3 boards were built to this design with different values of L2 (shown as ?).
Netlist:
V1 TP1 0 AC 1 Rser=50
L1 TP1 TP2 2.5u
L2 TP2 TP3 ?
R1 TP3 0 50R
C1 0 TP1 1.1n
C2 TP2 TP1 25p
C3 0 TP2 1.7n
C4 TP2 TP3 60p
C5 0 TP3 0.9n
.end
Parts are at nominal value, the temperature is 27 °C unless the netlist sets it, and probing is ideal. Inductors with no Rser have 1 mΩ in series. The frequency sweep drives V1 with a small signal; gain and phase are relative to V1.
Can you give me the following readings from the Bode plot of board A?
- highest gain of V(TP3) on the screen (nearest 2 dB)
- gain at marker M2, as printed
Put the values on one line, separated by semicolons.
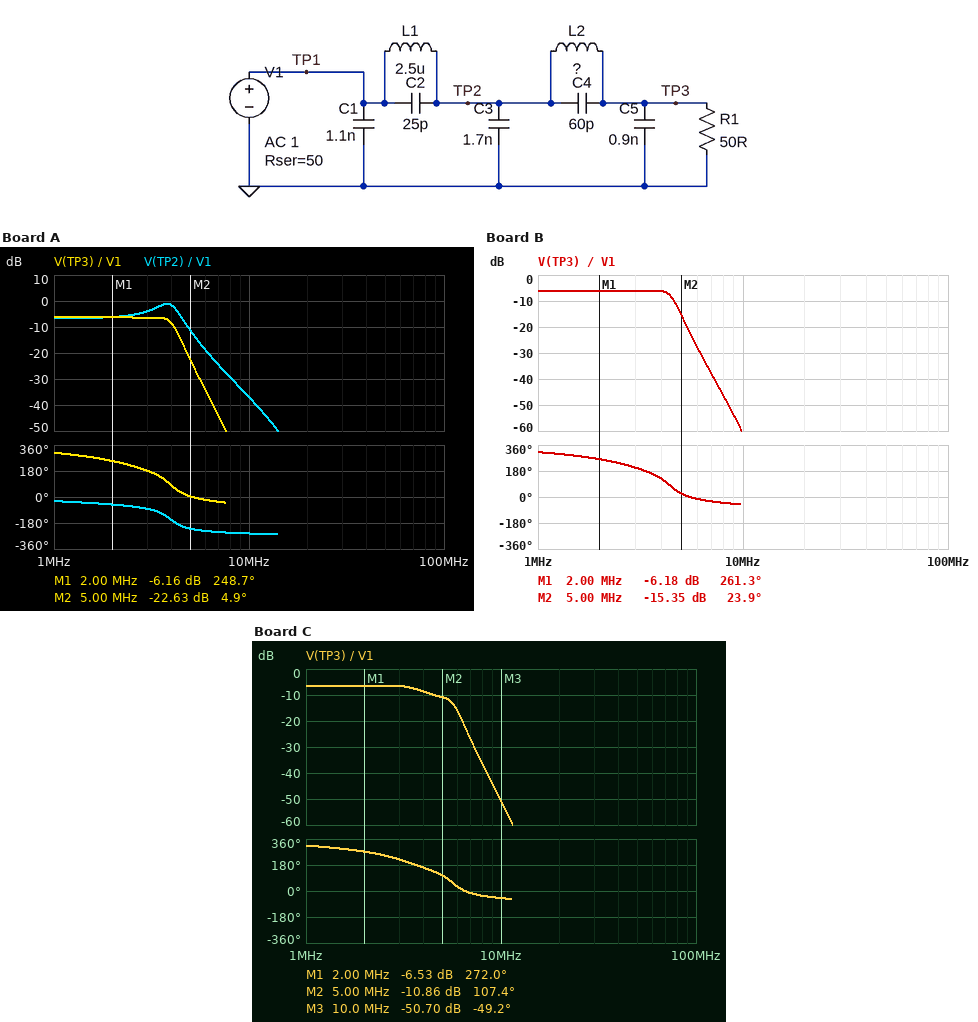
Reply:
-6 dB; -22.63 dB
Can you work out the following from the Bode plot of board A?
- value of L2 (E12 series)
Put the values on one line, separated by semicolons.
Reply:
3.3 µH
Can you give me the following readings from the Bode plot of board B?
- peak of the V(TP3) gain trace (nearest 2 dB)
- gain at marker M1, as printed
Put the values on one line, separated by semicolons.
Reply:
-6 dB; -6.18 dB
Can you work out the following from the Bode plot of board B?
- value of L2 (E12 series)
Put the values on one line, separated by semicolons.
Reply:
2.2 µH
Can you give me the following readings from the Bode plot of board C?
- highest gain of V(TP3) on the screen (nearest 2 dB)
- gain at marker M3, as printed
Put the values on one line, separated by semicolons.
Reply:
-6 dB; -50.70 dB
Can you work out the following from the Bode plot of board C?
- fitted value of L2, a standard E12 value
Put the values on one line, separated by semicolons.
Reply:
1.2 µH
